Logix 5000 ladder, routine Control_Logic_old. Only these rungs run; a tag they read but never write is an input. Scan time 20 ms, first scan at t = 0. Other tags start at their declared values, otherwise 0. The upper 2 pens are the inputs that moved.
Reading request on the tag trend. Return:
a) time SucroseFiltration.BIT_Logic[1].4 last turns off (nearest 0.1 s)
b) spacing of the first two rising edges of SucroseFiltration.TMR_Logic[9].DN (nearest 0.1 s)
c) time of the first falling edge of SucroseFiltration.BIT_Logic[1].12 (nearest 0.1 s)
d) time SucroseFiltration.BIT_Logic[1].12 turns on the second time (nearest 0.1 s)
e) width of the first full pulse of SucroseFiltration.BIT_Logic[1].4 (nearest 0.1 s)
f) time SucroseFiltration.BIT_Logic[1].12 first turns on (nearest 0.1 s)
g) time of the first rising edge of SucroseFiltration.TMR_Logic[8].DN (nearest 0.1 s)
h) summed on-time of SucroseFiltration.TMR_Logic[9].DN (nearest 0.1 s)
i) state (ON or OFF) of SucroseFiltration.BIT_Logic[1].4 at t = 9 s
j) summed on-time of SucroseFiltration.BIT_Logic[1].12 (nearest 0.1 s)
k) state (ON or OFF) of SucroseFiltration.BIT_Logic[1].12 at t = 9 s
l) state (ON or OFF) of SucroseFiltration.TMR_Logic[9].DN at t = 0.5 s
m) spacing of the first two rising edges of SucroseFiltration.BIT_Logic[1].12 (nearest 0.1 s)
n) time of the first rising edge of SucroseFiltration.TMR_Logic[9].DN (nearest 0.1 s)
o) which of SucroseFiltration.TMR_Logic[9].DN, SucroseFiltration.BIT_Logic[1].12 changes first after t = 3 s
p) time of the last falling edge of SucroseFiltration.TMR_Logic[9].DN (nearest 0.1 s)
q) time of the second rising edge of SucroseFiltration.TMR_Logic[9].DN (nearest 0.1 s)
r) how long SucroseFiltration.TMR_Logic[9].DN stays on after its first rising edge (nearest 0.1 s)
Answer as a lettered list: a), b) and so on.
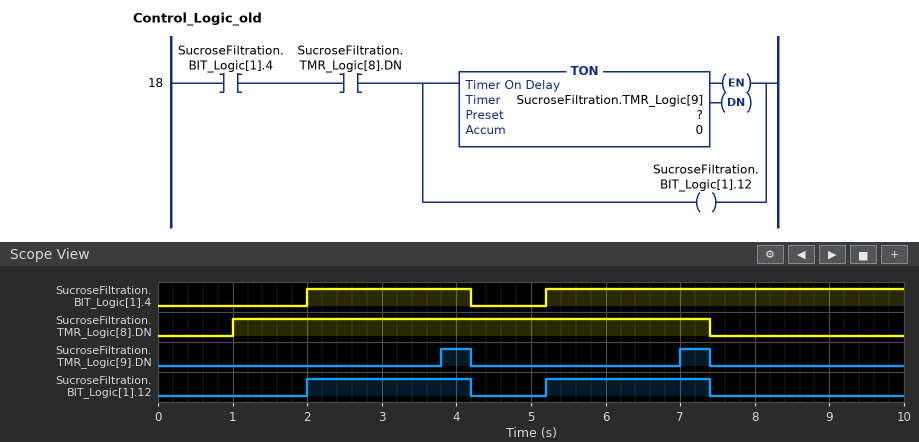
a) 4.2 s
b) 3.2 s
c) 4.2 s
d) 5.2 s
e) 2.2 s
f) 2.0 s
g) 1.0 s
h) 0.8 s
i) ON
j) 4.4 s
k) OFF
l) OFF
m) 3.2 s
n) 3.8 s
o) SucroseFiltration.TMR_Logic[9].DN
p) 7.4 s
q) 7.0 s
r) 0.4 s
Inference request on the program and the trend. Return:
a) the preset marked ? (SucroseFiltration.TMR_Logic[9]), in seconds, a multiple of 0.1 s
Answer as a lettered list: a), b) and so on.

a) 1.8 s
